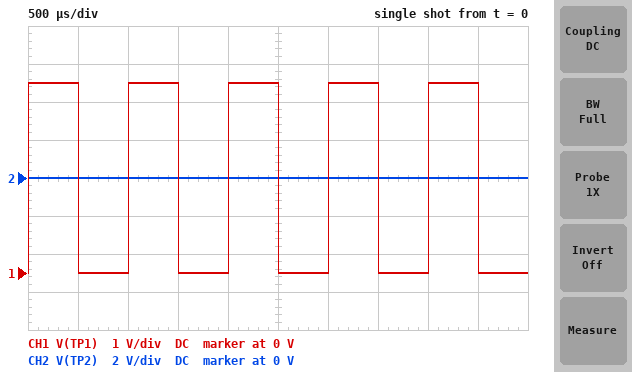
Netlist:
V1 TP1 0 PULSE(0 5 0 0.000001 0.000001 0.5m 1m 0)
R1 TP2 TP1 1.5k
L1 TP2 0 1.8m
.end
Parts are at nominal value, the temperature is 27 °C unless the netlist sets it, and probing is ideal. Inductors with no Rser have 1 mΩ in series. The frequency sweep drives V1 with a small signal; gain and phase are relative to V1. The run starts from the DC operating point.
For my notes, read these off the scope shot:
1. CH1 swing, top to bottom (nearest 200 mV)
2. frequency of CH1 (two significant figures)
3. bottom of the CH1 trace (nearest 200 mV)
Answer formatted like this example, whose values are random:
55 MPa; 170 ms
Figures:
5.0 V; 1.0 kHz; 0 V
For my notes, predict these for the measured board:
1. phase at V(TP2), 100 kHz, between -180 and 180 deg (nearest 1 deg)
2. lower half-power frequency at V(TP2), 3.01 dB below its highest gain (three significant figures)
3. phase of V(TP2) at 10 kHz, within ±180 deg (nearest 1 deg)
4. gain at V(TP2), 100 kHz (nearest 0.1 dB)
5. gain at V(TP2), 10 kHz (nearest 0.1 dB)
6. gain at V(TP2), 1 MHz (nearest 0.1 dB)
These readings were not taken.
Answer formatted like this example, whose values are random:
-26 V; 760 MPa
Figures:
53 deg; 133 kHz; 86 deg; -4.4 dB; -22.5 dB; -0.1 dB
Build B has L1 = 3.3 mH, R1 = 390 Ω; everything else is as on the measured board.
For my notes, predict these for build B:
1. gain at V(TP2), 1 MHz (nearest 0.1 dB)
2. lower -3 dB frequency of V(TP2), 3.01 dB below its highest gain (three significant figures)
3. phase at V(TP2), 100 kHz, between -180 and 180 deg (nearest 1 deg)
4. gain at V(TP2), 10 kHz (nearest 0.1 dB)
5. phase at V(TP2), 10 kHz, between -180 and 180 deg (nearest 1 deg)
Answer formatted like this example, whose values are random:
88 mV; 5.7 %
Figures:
0 dB; 18.8 kHz; 11 deg; -6.6 dB; 62 deg
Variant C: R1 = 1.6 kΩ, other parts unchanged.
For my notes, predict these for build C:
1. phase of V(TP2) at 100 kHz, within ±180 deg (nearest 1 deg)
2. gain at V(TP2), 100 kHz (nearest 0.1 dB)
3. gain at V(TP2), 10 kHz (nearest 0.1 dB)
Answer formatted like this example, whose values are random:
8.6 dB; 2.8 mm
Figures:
55 deg; -4.8 dB; -23.0 dB
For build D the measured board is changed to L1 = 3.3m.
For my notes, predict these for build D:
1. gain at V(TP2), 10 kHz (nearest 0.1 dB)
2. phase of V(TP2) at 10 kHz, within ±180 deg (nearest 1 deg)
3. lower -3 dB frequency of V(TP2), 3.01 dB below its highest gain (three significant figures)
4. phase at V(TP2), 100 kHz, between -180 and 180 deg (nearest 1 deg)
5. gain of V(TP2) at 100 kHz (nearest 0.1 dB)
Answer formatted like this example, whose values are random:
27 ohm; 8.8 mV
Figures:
-17.3 dB; 82 deg; 72.3 kHz; 36 deg; -1.8 dB
